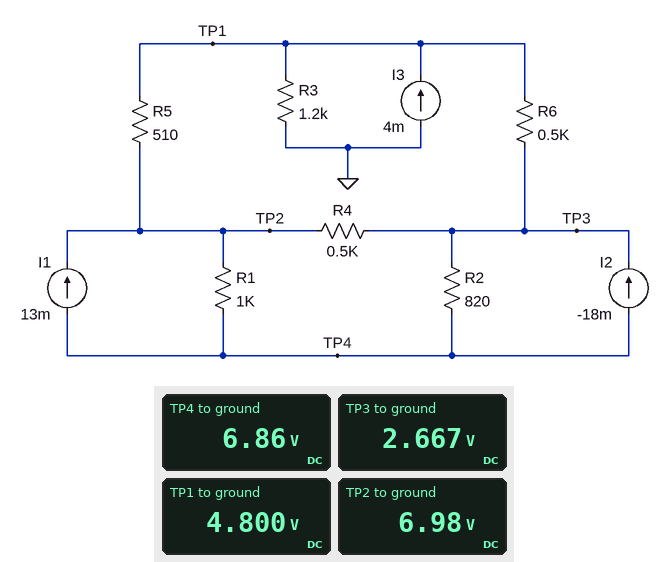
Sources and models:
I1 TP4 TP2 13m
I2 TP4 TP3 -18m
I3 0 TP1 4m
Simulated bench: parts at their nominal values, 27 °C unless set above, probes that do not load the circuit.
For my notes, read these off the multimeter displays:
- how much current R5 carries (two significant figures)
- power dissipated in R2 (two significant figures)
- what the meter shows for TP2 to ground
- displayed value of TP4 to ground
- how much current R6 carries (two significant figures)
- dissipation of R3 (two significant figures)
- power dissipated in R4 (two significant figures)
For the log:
4.3 mA
21 mW
6.98 V
6.86 V
4.3 mA
19 mW
37 mW
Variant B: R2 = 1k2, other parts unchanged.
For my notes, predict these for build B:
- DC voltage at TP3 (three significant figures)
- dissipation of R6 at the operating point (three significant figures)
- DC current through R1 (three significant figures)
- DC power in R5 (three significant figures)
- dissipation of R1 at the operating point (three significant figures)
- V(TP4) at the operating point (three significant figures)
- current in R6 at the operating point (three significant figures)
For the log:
2.54 V
10.2 mW
652 µA
10.4 mW
425 µW
7.76 V
4.52 mA
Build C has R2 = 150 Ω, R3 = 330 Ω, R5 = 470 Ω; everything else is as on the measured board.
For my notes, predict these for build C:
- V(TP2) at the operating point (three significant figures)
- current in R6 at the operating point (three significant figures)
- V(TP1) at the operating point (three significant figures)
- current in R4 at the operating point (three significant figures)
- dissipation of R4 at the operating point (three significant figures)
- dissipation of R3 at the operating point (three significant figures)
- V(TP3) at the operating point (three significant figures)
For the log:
3.02 V
3.61 mA
1.32 V
7.00 mA
24.5 mW
5.28 mW
-484 mV
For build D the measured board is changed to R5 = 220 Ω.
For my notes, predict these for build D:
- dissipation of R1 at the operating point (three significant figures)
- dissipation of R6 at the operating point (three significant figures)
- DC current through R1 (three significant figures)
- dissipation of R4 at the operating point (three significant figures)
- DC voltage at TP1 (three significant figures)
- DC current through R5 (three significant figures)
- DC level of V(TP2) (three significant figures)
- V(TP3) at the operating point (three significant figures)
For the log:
15.6 µW
14.5 mW
125 µA
30.0 mW
4.80 V
5.38 mA
5.98 V
2.11 V
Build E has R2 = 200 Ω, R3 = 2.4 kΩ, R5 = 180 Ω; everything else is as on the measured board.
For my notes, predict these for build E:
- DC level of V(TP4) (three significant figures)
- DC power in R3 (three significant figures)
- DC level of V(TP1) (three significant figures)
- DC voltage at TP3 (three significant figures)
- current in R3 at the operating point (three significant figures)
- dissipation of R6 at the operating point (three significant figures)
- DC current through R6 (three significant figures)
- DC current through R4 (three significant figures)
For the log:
8.61 V
38.4 mW
9.60 V
7.24 V
4.00 mA
11.2 mW
4.73 mA
6.43 mA
